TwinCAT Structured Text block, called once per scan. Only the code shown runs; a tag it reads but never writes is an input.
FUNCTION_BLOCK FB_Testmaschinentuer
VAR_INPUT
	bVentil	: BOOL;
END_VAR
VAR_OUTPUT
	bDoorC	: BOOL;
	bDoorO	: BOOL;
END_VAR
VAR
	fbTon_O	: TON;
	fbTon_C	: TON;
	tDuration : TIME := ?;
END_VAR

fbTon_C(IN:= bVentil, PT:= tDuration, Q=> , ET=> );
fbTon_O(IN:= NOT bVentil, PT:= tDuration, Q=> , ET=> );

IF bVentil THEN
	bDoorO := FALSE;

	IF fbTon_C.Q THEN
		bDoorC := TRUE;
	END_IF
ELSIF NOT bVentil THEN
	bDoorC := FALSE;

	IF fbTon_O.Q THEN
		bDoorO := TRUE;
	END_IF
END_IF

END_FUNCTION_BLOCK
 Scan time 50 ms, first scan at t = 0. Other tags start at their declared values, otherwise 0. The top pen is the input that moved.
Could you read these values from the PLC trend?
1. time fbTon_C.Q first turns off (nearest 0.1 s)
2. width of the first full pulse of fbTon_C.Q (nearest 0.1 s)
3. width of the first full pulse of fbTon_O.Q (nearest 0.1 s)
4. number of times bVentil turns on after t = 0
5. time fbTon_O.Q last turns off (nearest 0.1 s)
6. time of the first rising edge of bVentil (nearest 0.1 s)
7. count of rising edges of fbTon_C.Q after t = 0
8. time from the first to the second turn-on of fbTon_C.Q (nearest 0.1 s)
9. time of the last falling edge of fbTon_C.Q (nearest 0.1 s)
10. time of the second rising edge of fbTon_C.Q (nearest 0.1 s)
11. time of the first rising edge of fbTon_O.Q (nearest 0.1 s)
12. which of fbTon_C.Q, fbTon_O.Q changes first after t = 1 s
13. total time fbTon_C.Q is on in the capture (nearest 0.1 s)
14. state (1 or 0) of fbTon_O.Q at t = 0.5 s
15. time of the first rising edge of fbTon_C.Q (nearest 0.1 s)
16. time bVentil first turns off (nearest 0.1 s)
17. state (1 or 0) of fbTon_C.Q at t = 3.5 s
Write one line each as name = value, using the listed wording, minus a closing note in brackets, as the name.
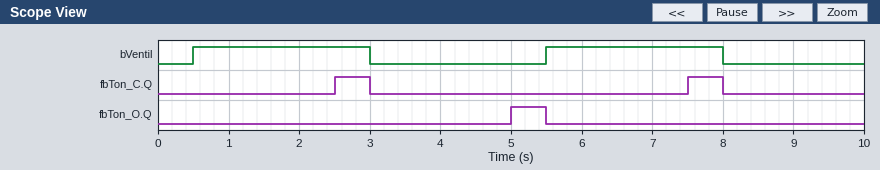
time fbTon_C.Q first turns off = 3.0 s
width of the first full pulse of fbTon_C.Q = 0.5 s
width of the first full pulse of fbTon_O.Q = 0.5 s
number of times bVentil turns on after t = 0 = 2
time fbTon_O.Q last turns off = 5.5 s
time of the first rising edge of bVentil = 0.5 s
count of rising edges of fbTon_C.Q after t = 0 = 2
time from the first to the second turn-on of fbTon_C.Q = 5.0 s
time of the last falling edge of fbTon_C.Q = 8.0 s
time of the second rising edge of fbTon_C.Q = 7.5 s
time of the first rising edge of fbTon_O.Q = 5.0 s
which of fbTon_C.Q, fbTon_O.Q changes first after t = 1 s = fbTon_C.Q
total time fbTon_C.Q is on in the capture = 1.0 s
state (1 or 0) of fbTon_O.Q at t = 0.5 s = 0
time of the first rising edge of fbTon_C.Q = 2.5 s
time bVentil first turns off = 3.0 s
state (1 or 0) of fbTon_C.Q at t = 3.5 s = 0
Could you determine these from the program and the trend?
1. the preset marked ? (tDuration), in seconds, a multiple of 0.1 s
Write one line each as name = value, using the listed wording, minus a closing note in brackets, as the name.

the preset marked ? (tDuration), in seconds, a multiple of 0.1 s = 2.0 s
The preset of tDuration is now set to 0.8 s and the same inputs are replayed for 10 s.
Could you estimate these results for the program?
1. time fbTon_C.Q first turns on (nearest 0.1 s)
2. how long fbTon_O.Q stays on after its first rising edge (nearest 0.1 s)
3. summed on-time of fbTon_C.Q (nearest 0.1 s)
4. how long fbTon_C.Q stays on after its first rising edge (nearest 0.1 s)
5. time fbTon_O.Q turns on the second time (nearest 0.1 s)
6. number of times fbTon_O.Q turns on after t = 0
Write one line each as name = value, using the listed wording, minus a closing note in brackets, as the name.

time fbTon_C.Q first turns on = 1.3 s
how long fbTon_O.Q stays on after its first rising edge = 1.7 s
summed on-time of fbTon_C.Q = 3.4 s
how long fbTon_C.Q stays on after its first rising edge = 1.7 s
time fbTon_O.Q turns on the second time = 8.8 s
number of times fbTon_O.Q turns on after t = 0 = 2
